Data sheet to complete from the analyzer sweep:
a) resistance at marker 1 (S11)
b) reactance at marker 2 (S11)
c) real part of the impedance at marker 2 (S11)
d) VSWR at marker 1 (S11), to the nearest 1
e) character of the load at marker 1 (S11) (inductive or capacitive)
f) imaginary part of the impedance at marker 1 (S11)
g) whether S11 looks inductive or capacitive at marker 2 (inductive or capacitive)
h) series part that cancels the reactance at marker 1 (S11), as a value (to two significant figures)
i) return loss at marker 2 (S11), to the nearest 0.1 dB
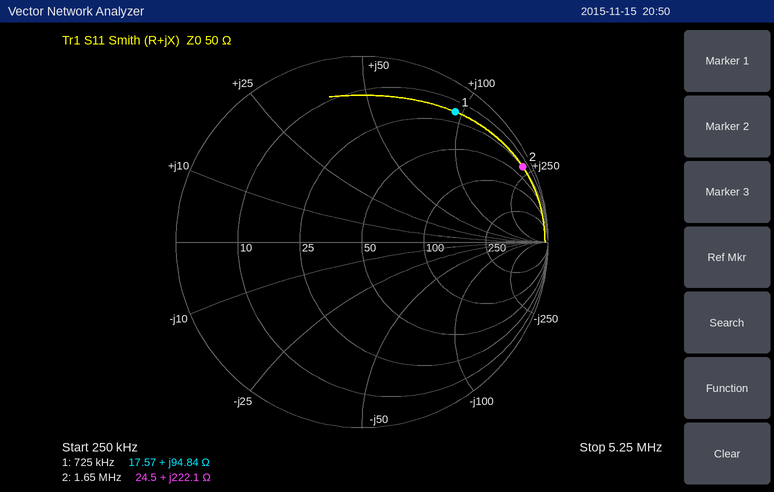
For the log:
17.57 Ω
+222.1 Ω
24.5 Ω
13
inductive
+94.84 Ω
inductive
2.3 nF
0.4 dB
